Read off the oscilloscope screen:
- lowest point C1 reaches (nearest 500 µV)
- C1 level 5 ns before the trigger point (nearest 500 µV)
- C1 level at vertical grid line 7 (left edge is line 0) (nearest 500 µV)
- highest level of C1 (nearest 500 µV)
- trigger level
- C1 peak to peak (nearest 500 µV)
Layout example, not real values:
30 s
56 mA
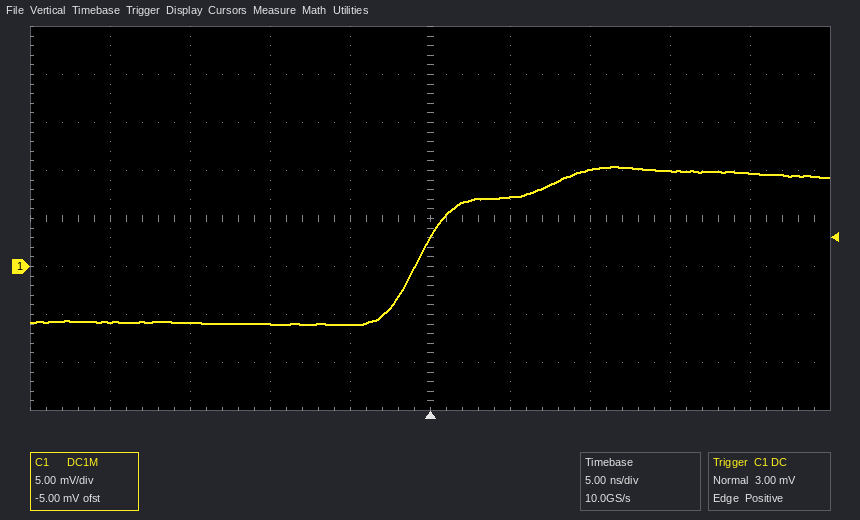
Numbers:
-6.0 mV
-6.0 mV
10.0 mV
10.5 mV
3.00 mV
16.5 mV
